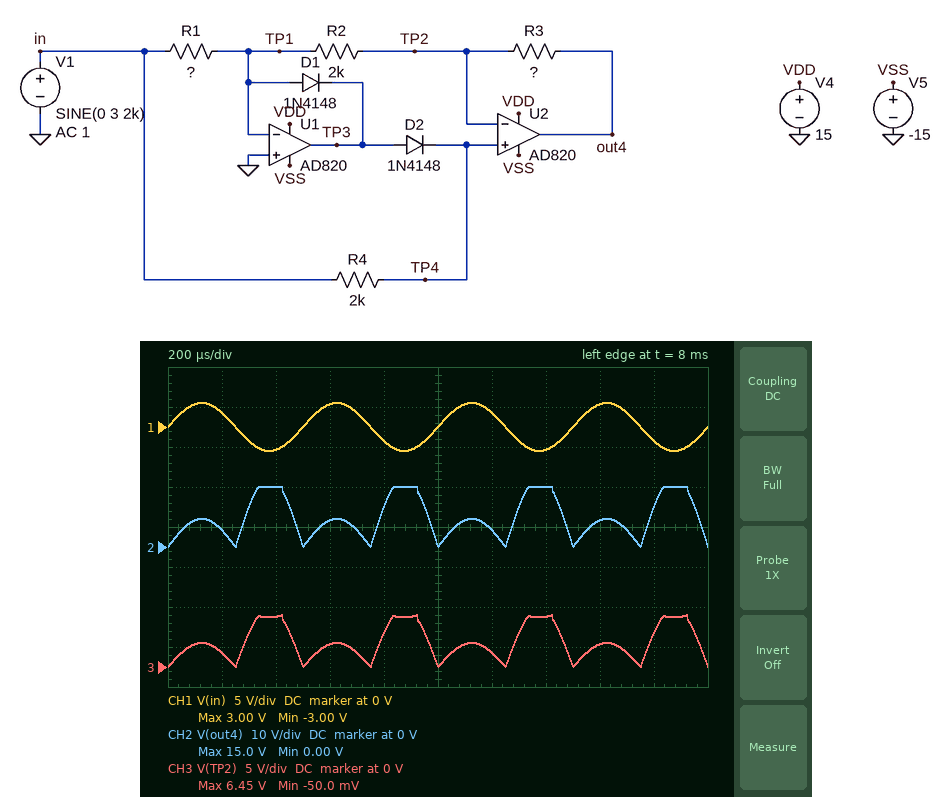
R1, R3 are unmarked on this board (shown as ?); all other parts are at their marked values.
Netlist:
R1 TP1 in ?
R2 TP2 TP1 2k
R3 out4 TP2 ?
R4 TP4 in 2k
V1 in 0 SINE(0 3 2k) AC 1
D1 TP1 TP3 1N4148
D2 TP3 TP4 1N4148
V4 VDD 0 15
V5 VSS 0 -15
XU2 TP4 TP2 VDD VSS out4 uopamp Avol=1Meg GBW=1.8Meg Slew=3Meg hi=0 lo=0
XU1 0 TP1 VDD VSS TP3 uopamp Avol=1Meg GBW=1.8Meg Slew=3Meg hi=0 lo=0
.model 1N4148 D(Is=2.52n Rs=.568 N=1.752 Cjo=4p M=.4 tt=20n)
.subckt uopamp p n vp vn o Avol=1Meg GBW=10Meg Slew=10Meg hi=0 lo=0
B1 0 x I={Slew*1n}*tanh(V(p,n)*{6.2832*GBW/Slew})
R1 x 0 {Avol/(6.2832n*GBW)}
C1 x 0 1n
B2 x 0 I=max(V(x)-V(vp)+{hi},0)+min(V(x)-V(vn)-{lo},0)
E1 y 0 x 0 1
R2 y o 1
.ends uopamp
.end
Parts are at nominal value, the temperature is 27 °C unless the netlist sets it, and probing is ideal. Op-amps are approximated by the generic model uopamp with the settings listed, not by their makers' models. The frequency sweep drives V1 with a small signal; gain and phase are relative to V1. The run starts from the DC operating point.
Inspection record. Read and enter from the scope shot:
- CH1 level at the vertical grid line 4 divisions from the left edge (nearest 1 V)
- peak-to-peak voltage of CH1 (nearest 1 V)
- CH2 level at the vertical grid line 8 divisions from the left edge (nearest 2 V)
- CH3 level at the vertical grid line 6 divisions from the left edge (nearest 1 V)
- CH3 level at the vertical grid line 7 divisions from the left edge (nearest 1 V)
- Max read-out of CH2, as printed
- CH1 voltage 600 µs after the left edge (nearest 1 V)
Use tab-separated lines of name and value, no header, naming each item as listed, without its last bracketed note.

CH1 level at the vertical grid line 4 divisions from the left edge	-2 V
peak-to-peak voltage of CH1	6 V
CH2 level at the vertical grid line 8 divisions from the left edge	6 V
CH3 level at the vertical grid line 6 divisions from the left edge	2 V
CH3 level at the vertical grid line 7 divisions from the left edge	6 V
Max read-out of CH2, as printed	15.0 V
CH1 voltage 600 µs after the left edge	3 V
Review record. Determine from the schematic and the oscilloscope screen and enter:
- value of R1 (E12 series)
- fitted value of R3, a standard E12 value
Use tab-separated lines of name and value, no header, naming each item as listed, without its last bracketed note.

value of R1	820 Ω
fitted value of R3, a standard E12 value	2.7 kΩ
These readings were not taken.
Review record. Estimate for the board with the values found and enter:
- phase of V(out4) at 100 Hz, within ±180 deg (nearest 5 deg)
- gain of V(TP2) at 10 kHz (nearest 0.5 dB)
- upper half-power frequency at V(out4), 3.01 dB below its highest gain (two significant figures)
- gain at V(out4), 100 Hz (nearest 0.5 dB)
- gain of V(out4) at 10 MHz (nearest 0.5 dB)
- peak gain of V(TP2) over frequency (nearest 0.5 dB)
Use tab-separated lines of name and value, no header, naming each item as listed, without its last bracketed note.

phase of V(out4) at 100 Hz, within ±180 deg	115 deg
gain of V(TP2) at 10 kHz	-1.0 dB
upper half-power frequency at V(out4), 3.01 dB below its highest gain	170 Hz
gain at V(out4), 100 Hz	2.5 dB
gain of V(out4) at 10 MHz	-23.0 dB
peak gain of V(TP2) over frequency	-1.0 dB
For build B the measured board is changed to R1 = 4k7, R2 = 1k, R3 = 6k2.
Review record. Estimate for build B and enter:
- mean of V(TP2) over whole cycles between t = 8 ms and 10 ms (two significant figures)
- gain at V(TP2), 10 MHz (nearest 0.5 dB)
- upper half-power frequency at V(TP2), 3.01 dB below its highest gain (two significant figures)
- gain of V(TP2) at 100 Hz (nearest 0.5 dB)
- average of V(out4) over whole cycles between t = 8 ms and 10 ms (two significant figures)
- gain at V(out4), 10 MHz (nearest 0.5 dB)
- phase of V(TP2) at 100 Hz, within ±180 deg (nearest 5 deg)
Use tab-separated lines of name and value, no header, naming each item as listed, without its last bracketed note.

mean of V(TP2) over whole cycles between t = 8 ms and 10 ms	1.0 V
gain at V(TP2), 10 MHz	-8.0 dB
upper half-power frequency at V(TP2), 3.01 dB below its highest gain	1.2 MHz
gain of V(TP2) at 100 Hz	-7.5 dB
average of V(out4) over whole cycles between t = 8 ms and 10 ms	7.2 V
gain at V(out4), 10 MHz	-21.0 dB
phase of V(TP2) at 100 Hz, within ±180 deg	40 deg
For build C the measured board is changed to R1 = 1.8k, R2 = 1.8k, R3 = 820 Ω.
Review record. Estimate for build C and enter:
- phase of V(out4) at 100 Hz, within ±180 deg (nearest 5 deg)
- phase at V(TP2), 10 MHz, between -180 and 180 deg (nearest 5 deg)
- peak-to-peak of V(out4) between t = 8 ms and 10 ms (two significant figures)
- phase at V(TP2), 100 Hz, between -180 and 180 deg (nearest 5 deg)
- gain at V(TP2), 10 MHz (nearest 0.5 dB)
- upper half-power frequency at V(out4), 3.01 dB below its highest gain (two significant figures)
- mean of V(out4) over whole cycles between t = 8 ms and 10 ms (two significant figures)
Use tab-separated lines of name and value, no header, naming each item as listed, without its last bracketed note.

phase of V(out4) at 100 Hz, within ±180 deg	70 deg
phase at V(TP2), 10 MHz, between -180 and 180 deg	-45 deg
peak-to-peak of V(out4) between t = 8 ms and 10 ms	4.4 V
phase at V(TP2), 100 Hz, between -180 and 180 deg	65 deg
gain at V(TP2), 10 MHz	-14.5 dB
upper half-power frequency at V(out4), 3.01 dB below its highest gain	1.5 MHz
mean of V(out4) over whole cycles between t = 8 ms and 10 ms	2.8 V
